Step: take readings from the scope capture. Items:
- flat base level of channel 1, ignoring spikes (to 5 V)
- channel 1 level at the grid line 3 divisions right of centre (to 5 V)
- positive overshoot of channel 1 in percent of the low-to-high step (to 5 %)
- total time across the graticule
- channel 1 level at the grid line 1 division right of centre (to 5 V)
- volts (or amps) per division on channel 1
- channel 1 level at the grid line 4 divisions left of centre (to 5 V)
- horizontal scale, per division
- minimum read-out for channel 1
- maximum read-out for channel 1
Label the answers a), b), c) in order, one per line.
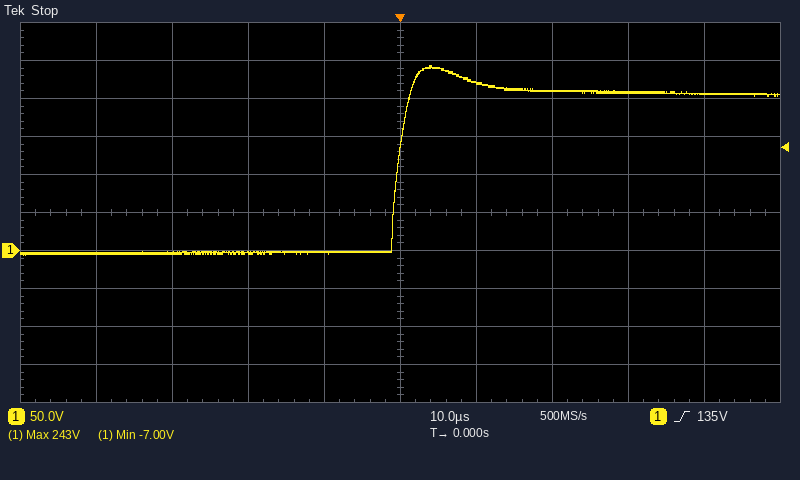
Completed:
a) -5 V
b) 210 V
c) 15 %
d) 100 µs
e) 220 V
f) 50 V
g) -5 V
h) 10 µs
i) -7.00 V
j) 243 V
